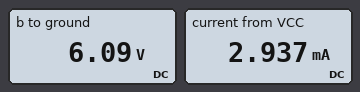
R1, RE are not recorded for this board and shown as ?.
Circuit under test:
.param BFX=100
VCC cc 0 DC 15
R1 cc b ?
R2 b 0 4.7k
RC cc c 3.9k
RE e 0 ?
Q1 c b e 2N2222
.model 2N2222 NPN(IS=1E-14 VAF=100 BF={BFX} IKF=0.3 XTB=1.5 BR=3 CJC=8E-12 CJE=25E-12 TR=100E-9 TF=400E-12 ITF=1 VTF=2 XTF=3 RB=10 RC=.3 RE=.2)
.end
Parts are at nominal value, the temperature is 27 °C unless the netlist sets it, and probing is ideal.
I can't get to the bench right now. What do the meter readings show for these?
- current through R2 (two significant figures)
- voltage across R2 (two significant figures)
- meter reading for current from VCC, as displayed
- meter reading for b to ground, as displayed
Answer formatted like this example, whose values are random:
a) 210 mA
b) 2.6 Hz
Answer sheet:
a) 1.3 mA
b) 6.1 V
c) 2.937 mA
d) 6.09 V
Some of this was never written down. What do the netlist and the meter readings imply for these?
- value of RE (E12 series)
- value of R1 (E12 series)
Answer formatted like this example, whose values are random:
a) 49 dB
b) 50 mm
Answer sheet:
a) 3.3 kΩ
b) 6.8 kΩ
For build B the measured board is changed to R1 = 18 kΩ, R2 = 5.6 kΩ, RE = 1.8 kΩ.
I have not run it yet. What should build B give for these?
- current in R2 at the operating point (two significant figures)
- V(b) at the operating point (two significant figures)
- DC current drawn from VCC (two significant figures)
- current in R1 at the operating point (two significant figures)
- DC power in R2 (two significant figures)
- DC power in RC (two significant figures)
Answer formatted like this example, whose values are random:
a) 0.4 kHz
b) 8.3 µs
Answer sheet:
a) 620 µA
b) 3.5 V
c) 2.2 mA
d) 640 µA
e) 2.2 mW
f) 9.5 mW
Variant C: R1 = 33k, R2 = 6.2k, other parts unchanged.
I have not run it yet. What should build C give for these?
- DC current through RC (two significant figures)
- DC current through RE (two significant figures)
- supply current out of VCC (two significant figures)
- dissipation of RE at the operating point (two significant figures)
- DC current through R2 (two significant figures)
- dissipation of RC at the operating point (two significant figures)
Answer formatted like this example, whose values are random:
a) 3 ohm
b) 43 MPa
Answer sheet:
a) 510 µA
b) 520 µA
c) 900 µA
d) 890 µW
e) 380 µA
f) 1.0 mW
